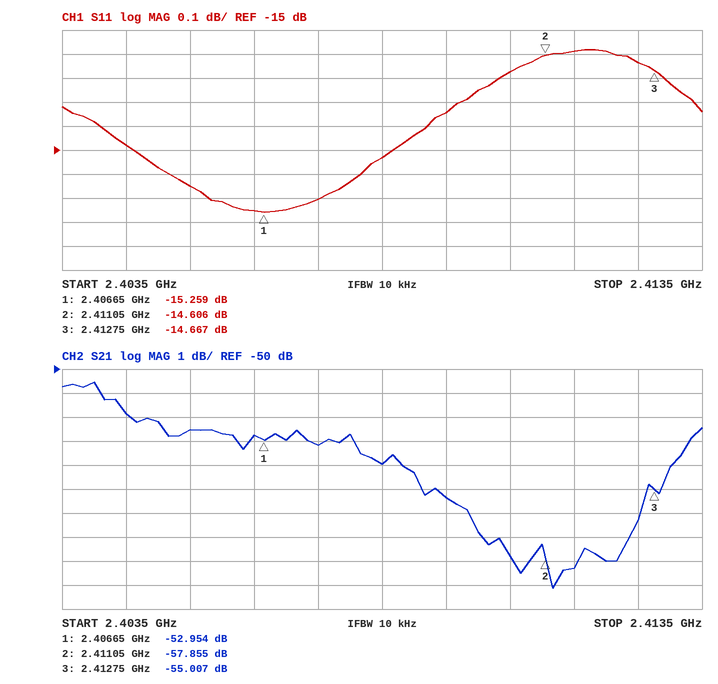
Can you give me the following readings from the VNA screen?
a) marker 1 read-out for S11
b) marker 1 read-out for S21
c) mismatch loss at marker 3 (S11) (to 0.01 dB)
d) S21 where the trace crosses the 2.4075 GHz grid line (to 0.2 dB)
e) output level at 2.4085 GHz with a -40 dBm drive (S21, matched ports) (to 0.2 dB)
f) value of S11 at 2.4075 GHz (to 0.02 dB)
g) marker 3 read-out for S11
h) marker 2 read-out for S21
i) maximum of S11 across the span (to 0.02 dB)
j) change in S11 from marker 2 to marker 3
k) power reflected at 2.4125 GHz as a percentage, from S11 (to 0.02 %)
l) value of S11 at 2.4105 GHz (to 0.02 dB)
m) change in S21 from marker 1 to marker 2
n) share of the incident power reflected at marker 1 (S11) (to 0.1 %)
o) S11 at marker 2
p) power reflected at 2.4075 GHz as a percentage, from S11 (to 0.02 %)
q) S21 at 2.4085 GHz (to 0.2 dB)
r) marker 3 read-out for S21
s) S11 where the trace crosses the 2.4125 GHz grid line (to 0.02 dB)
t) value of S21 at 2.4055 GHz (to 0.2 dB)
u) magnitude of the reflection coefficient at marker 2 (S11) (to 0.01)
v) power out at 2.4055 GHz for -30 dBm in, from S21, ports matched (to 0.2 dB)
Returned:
-15.259 dB
-52.954 dB
0.15 dB
-53.2 dB
-94.0 dBm
-15.20 dB
-14.667 dB
-57.855 dB
-14.58 dB
-0.061 dB
3.44 %
-14.68 dB
-4.901 dB
3.0 %
-14.606 dB
3.02 %
-54.0 dB
-55.007 dB
-14.64 dB
-52.6 dB
0.19
-82.6 dBm
